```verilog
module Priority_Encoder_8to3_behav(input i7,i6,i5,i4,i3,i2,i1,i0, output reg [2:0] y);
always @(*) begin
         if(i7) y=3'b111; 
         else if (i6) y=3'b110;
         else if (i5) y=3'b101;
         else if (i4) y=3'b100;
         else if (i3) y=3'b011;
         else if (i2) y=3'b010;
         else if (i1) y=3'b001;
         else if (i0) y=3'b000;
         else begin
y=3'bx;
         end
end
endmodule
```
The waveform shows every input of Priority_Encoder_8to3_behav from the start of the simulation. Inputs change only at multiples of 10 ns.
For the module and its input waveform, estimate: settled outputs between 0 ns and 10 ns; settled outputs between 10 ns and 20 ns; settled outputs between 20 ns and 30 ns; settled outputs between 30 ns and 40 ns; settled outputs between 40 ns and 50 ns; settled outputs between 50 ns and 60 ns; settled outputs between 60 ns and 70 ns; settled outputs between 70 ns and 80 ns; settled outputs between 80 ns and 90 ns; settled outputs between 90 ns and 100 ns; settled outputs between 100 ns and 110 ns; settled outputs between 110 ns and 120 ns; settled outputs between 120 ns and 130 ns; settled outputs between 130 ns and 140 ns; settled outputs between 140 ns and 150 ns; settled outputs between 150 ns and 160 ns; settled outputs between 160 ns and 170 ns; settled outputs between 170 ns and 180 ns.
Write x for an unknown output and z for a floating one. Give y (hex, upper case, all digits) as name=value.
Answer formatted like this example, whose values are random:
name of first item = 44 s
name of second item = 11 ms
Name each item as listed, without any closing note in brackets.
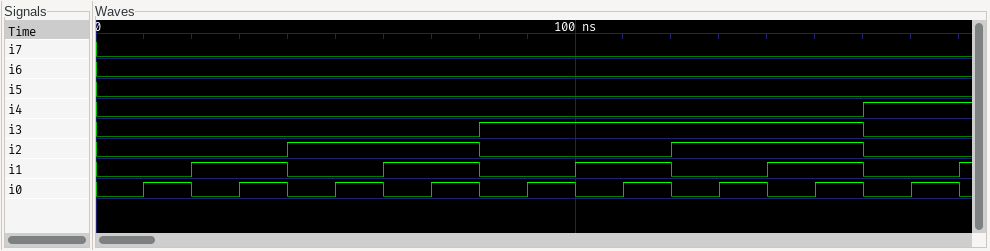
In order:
settled outputs between 0 ns and 10 ns = y=x
settled outputs between 10 ns and 20 ns = y=0
settled outputs between 20 ns and 30 ns = y=1
settled outputs between 30 ns and 40 ns = y=1
settled outputs between 40 ns and 50 ns = y=2
settled outputs between 50 ns and 60 ns = y=2
settled outputs between 60 ns and 70 ns = y=2
settled outputs between 70 ns and 80 ns = y=2
settled outputs between 80 ns and 90 ns = y=3
settled outputs between 90 ns and 100 ns = y=3
settled outputs between 100 ns and 110 ns = y=3
settled outputs between 110 ns and 120 ns = y=3
settled outputs between 120 ns and 130 ns = y=3
settled outputs between 130 ns and 140 ns = y=3
settled outputs between 140 ns and 150 ns = y=3
settled outputs between 150 ns and 160 ns = y=3
settled outputs between 160 ns and 170 ns = y=4
settled outputs between 170 ns and 180 ns = y=4
